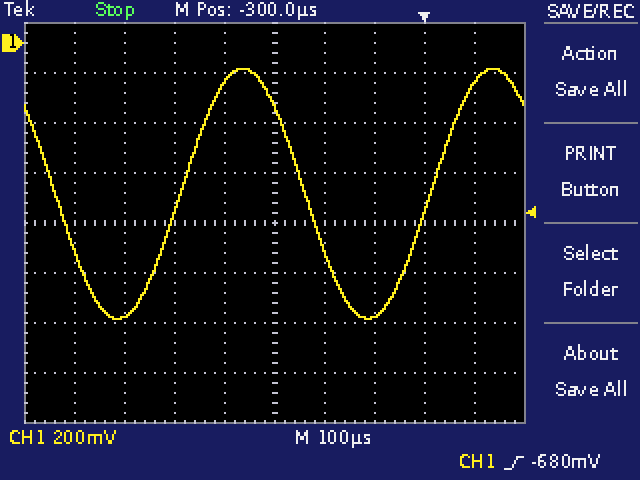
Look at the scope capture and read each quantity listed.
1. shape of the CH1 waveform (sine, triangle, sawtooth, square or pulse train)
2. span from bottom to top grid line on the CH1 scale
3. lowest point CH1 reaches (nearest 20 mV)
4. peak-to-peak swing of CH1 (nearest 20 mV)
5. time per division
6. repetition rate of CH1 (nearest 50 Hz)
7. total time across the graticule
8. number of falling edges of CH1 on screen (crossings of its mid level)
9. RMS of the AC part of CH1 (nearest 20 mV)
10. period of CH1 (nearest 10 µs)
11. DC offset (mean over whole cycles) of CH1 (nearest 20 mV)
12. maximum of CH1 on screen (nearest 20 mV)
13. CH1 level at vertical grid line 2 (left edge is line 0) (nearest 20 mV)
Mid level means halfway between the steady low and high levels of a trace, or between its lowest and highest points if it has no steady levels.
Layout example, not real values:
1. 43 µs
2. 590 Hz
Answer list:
1. sine
2. 1.6 V
3. -1.10 V
4. 1.00 V
5. 100 µs
6. 2.00 kHz
7. 1 ms
8. 2
9. 360 mV
10. 500 µs
11. -600 mV
12. -100 mV
13. -1.10 V
